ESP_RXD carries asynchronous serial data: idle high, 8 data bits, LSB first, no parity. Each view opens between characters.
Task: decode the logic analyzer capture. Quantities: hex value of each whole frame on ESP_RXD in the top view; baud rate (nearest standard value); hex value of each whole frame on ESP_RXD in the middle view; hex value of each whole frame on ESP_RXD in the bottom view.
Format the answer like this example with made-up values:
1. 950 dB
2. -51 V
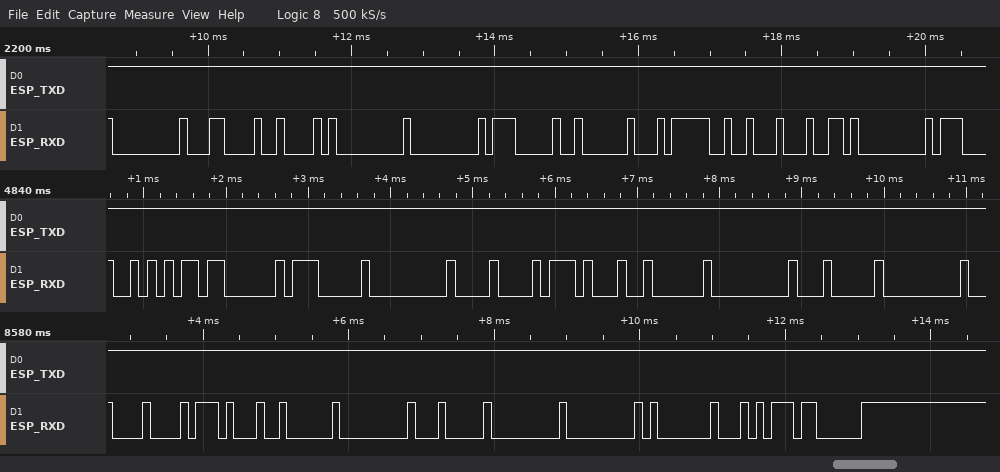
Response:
1. 00, 0C, 42, 00, 00, 07, 02, F4, 12, 64, 00
2. 9600 baud
3. AA, 03, 07, 00, 08, 17, 02, 00, 04, 00
4. 08, 17, 02, 00, 04, 00, 00, 01, D4, 03
